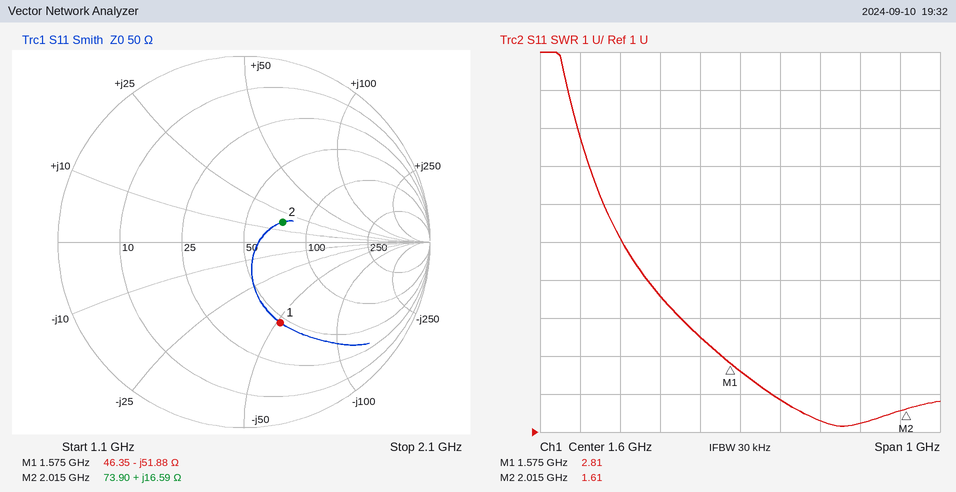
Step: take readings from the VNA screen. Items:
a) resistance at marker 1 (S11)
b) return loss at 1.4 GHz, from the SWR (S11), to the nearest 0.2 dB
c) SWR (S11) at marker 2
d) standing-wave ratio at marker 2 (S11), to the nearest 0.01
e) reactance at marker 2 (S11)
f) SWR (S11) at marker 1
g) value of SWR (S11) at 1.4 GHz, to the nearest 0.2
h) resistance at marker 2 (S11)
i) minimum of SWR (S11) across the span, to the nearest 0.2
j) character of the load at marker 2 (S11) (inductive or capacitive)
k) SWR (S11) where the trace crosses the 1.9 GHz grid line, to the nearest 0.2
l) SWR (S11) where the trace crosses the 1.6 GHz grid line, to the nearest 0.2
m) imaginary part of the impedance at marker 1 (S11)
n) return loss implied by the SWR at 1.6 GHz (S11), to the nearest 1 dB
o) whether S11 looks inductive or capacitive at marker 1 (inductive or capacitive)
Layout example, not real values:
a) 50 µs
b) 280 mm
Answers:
a) 46.35 Ω
b) 3.8 dB
c) 1.61
d) 1.61
e) +16.59 Ω
f) 2.81
g) 4.6
h) 73.90 Ω
i) 1.2
j) inductive
k) 1.2
l) 2.6
m) -51.88 Ω
n) 7 dB
o) capacitive
